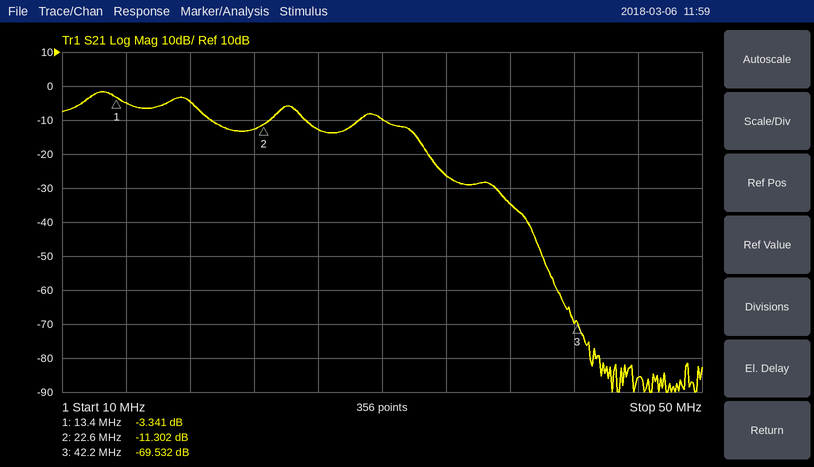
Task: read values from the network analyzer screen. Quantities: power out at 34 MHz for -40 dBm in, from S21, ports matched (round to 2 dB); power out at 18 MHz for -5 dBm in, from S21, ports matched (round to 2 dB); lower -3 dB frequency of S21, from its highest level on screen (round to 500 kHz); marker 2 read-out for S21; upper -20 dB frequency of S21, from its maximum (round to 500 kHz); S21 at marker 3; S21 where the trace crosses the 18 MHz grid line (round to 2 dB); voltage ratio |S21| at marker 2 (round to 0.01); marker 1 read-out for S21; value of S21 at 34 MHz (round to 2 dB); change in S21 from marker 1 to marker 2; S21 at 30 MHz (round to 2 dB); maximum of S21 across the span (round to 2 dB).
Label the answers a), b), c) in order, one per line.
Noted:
a) -66 dBm
b) -10 dBm
c) 11.5 MHz
d) -11.302 dB
e) 33.0 MHz
f) -69.532 dB
g) -4 dB
h) 0.27
i) -3.341 dB
j) -26 dB
k) -7.961 dB
l) -10 dB
m) -2 dB
